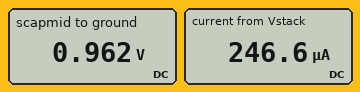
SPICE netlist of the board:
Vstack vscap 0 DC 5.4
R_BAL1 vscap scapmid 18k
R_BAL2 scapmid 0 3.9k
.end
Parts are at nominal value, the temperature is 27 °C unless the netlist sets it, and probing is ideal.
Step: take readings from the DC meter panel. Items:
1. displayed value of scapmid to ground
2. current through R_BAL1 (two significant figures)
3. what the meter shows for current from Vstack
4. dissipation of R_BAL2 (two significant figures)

0.962 V
250 µA
246.6 µA
240 µW
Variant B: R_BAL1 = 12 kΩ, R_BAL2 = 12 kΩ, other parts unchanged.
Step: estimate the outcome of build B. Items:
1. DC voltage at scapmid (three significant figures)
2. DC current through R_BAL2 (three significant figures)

2.70 V
225 µA
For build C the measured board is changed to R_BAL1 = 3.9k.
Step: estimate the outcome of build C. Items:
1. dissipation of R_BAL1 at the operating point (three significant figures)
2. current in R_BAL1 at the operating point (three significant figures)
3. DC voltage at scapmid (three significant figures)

1.87 mW
692 µA
2.70 V
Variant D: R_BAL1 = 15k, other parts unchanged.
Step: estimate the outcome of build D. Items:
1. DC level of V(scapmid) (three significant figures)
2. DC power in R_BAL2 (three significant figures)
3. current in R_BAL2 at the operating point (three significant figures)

1.11 V
318 µW
286 µA
